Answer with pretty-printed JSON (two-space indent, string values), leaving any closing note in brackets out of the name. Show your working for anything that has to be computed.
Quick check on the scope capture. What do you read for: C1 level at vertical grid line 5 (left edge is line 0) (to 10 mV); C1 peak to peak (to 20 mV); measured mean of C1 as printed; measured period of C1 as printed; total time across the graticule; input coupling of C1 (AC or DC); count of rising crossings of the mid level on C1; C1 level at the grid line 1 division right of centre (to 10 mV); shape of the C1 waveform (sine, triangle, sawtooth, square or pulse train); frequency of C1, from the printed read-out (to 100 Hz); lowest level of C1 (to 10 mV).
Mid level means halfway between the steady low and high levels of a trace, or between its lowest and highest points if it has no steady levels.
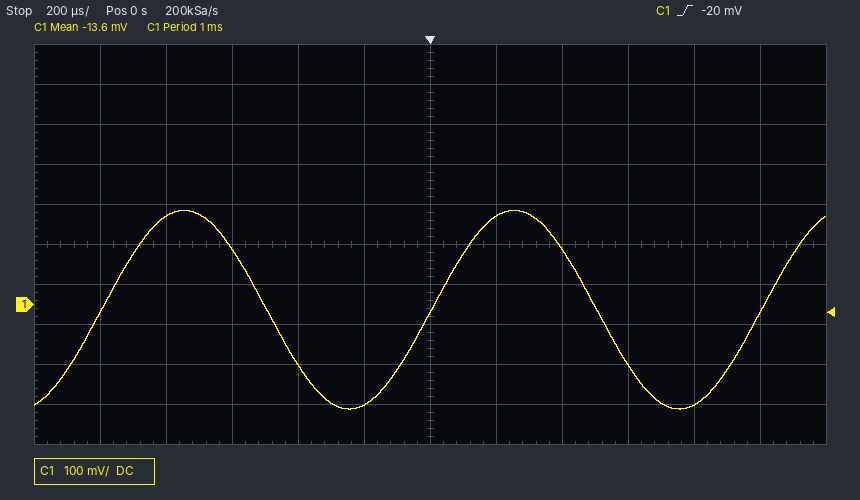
{
  "C1 level at vertical grid line 5 (left edge is line 0)": "-250 mV",
  "C1 peak to peak": "500 mV",
  "measured mean of C1 as printed": "-13.6 mV",
  "measured period of C1 as printed": "1 ms",
  "total time across the graticule": "2.4 ms",
  "input coupling of C1": "DC",
  "count of rising crossings of the mid level on C1": "3",
  "C1 level at the grid line 1 division right of centre": "220 mV",
  "shape of the C1 waveform": "sine",
  "frequency of C1, from the printed read-out": "1 / 1 ms ≈ 1.0 kHz",
  "lowest level of C1": "-260 mV"
}
